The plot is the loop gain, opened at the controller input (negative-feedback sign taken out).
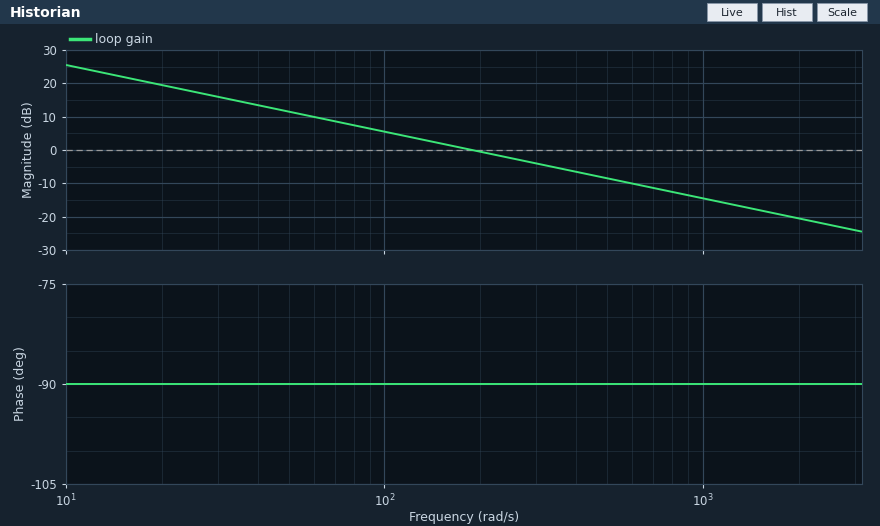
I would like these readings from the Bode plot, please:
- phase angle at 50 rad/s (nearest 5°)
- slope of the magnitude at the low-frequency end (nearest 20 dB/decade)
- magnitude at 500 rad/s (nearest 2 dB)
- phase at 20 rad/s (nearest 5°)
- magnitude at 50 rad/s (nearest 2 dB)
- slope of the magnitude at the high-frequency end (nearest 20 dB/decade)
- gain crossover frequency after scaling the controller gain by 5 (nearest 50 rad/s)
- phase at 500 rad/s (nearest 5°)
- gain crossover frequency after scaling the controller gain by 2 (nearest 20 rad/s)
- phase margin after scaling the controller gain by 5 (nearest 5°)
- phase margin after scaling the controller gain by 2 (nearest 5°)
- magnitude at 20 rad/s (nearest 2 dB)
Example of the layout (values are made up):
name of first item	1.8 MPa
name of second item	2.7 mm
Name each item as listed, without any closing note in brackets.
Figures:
phase angle at 50 rad/s	-90°
slope of the magnitude at the low-frequency end	-20 dB/decade
magnitude at 500 rad/s	-8 dB
phase at 20 rad/s	-90°
magnitude at 50 rad/s	12 dB
slope of the magnitude at the high-frequency end	-20 dB/decade
gain crossover frequency after scaling the controller gain by 5	950 rad/s
phase at 500 rad/s	-90°
gain crossover frequency after scaling the controller gain by 2	380 rad/s
phase margin after scaling the controller gain by 5	90°
phase margin after scaling the controller gain by 2	90°
magnitude at 20 rad/s	20 dB
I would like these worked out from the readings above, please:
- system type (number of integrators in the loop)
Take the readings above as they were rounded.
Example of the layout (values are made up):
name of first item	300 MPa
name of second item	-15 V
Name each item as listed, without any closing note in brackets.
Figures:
system type	1
